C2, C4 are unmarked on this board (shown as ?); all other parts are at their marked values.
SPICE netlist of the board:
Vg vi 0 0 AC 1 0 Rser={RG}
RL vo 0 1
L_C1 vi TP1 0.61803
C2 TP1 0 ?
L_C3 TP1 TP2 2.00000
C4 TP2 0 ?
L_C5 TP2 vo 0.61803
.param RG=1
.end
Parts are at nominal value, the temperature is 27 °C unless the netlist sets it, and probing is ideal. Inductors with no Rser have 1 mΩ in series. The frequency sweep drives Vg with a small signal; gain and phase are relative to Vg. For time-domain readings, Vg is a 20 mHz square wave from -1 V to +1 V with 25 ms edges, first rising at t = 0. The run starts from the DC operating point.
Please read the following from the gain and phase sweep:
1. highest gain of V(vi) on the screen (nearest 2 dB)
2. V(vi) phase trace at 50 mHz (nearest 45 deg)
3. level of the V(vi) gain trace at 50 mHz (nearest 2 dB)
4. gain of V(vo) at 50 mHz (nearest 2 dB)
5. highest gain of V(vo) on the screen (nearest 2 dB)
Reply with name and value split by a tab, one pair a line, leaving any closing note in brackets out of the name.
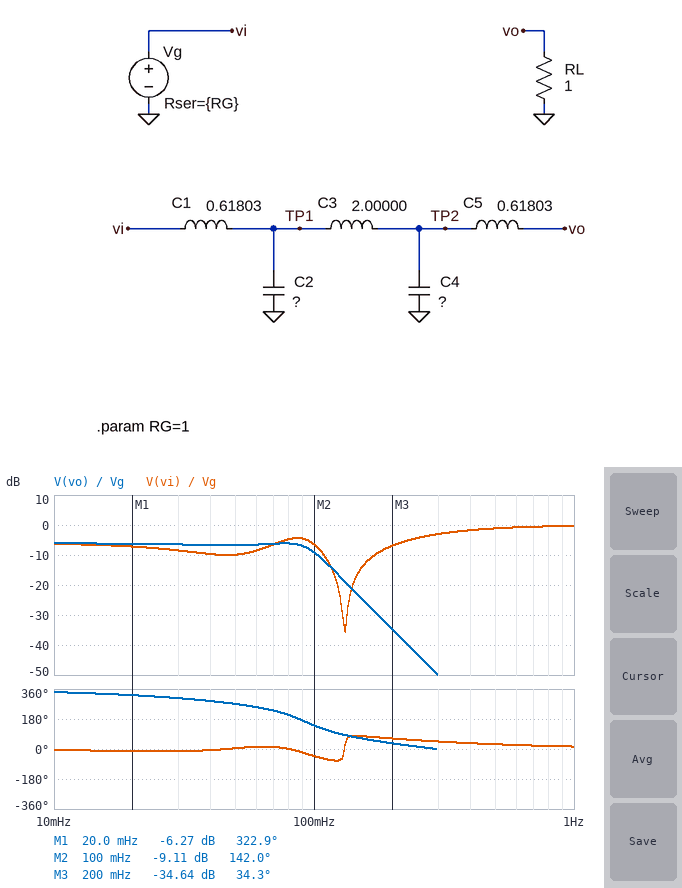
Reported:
highest gain of V(vi) on the screen	0 dB
V(vi) phase trace at 50 mHz	0 deg
level of the V(vi) gain trace at 50 mHz	-10 dB
gain of V(vo) at 50 mHz	-6 dB
highest gain of V(vo) on the screen	-6 dB
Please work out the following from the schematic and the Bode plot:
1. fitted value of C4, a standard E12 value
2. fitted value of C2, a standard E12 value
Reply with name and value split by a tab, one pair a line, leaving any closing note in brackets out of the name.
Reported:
fitted value of C4, a standard E12 value	3.9 F
fitted value of C2, a standard E12 value	3.3 F
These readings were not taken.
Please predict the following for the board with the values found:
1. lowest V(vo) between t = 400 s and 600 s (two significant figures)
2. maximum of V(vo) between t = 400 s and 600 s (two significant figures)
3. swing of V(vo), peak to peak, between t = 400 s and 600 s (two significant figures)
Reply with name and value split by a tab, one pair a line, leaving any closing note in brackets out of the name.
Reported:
lowest V(vo) between t = 400 s and 600 s	-590 mV
maximum of V(vo) between t = 400 s and 600 s	590 mV
swing of V(vo), peak to peak, between t = 400 s and 600 s	1.2 V
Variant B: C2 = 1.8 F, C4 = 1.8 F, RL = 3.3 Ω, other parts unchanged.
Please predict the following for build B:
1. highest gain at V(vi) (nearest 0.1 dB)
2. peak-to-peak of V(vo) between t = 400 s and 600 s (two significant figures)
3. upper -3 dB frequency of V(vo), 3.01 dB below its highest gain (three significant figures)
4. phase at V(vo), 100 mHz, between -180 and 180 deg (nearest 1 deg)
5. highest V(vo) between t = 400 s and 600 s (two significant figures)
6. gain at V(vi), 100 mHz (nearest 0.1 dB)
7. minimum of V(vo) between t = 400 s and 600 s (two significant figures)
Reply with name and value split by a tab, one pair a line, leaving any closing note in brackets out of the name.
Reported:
highest gain at V(vi)	0 dB
peak-to-peak of V(vo) between t = 400 s and 600 s	1.9 V
upper -3 dB frequency of V(vo), 3.01 dB below its highest gain	138 mHz
phase at V(vo), 100 mHz, between -180 and 180 deg	-134 deg
highest V(vo) between t = 400 s and 600 s	960 mV
gain at V(vi), 100 mHz	-4.9 dB
minimum of V(vo) between t = 400 s and 600 s	-960 mV
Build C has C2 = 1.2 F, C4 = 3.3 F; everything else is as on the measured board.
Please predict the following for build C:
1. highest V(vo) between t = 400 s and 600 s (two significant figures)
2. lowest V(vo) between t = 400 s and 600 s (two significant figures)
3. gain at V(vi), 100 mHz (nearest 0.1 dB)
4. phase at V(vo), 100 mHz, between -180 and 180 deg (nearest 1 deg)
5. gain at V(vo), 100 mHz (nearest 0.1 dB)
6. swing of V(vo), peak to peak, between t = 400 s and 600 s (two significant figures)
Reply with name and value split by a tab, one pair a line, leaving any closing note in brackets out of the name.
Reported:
highest V(vo) between t = 400 s and 600 s	550 mV
lowest V(vo) between t = 400 s and 600 s	-550 mV
gain at V(vi), 100 mHz	-2.3 dB
phase at V(vo), 100 mHz, between -180 and 180 deg	-148 deg
gain at V(vo), 100 mHz	-8.4 dB
swing of V(vo), peak to peak, between t = 400 s and 600 s	1.1 V
